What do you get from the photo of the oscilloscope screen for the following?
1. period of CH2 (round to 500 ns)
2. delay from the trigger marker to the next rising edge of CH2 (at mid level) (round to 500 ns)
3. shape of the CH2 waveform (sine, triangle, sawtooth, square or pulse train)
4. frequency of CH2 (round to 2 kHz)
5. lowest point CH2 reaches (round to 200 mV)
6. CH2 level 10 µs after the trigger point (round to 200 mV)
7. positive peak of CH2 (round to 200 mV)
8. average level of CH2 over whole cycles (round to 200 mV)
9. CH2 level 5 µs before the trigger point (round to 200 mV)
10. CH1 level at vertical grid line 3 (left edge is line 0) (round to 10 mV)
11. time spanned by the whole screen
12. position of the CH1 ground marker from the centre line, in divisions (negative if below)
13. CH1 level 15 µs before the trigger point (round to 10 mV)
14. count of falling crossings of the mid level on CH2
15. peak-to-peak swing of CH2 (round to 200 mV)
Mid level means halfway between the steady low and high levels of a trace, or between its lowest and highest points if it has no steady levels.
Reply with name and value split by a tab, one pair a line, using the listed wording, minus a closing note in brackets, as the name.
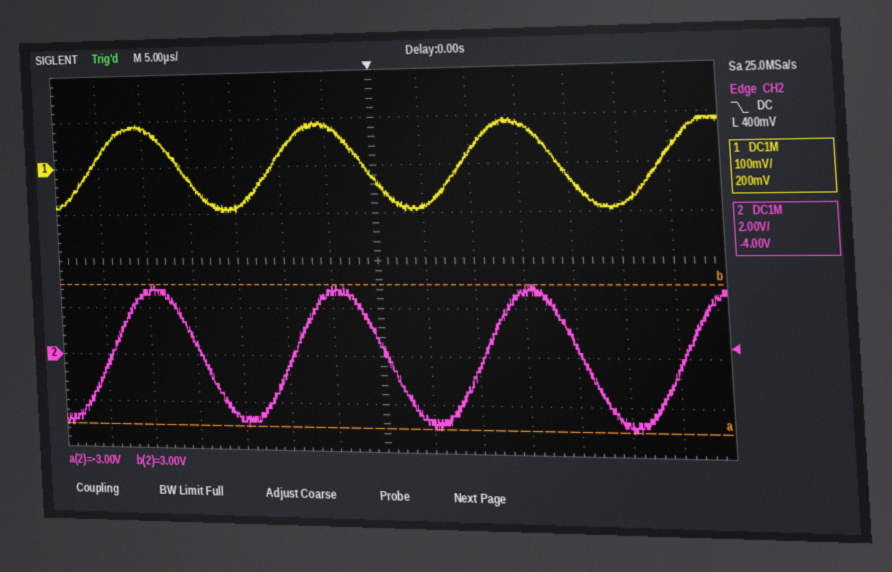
period of CH2	20.0 µs
delay from the trigger marker to the next rising edge of CH2 (at mid level)	10.5 µs
shape of the CH2 waveform	sine
frequency of CH2	50 kHz
lowest point CH2 reaches	-3.0 V
CH2 level 10 µs after the trigger point	-400 mV
positive peak of CH2	3.0 V
average level of CH2 over whole cycles	0.0 V
CH2 level 5 µs before the trigger point	2.8 V
CH1 level at vertical grid line 3 (left edge is line 0)	-20 mV
time spanned by the whole screen	70 µs
position of the CH1 ground marker from the centre line, in divisions	+2.0 div
CH1 level 15 µs before the trigger point	-90 mV
count of falling crossings of the mid level on CH2	3
peak-to-peak swing of CH2	6.0 V
